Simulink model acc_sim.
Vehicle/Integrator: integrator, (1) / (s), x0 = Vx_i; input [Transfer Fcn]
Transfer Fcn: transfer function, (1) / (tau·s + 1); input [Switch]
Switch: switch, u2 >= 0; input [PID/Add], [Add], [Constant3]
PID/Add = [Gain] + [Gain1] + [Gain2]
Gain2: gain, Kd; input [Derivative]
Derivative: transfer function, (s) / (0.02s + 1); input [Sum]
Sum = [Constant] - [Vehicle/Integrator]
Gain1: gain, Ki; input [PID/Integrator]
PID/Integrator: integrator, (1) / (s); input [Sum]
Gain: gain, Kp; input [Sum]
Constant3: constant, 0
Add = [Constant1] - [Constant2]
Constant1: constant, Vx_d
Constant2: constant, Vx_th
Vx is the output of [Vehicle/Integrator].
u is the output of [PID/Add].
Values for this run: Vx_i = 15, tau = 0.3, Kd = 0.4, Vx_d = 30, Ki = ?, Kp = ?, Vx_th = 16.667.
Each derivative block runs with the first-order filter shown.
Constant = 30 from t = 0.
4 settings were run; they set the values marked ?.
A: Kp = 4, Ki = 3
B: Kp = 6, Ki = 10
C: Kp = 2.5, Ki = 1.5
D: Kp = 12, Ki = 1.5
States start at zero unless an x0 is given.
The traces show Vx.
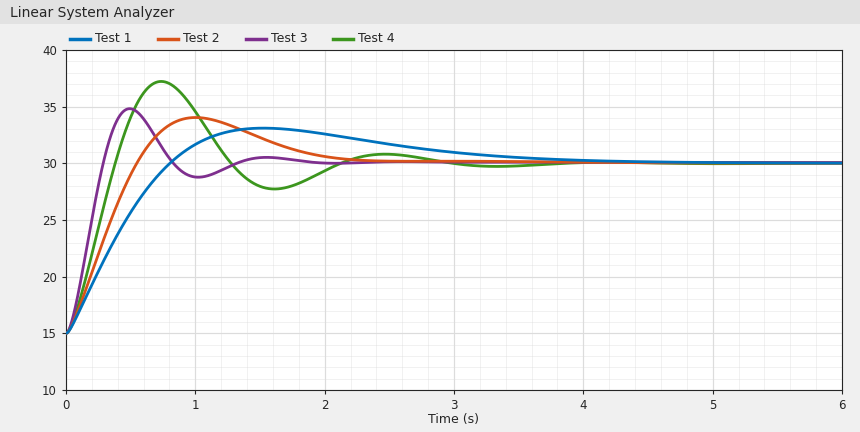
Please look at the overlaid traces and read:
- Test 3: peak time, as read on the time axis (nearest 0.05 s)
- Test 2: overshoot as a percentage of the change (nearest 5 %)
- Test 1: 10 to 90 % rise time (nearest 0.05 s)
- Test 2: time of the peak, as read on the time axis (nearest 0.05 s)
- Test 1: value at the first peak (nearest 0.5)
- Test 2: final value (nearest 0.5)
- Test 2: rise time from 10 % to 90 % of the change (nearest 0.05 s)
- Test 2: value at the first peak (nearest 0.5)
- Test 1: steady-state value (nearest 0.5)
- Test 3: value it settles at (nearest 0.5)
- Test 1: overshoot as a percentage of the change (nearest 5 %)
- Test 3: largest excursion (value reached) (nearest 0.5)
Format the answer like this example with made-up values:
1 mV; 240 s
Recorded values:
0.50 s; 25 %; 0.60 s; 1.00 s; 33.0; 30.0; 0.40 s; 34.0; 30.0; 30.0; 20 %; 35.0
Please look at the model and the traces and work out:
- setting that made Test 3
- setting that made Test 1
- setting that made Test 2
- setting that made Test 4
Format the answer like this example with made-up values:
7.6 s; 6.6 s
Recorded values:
D; C; A; B
